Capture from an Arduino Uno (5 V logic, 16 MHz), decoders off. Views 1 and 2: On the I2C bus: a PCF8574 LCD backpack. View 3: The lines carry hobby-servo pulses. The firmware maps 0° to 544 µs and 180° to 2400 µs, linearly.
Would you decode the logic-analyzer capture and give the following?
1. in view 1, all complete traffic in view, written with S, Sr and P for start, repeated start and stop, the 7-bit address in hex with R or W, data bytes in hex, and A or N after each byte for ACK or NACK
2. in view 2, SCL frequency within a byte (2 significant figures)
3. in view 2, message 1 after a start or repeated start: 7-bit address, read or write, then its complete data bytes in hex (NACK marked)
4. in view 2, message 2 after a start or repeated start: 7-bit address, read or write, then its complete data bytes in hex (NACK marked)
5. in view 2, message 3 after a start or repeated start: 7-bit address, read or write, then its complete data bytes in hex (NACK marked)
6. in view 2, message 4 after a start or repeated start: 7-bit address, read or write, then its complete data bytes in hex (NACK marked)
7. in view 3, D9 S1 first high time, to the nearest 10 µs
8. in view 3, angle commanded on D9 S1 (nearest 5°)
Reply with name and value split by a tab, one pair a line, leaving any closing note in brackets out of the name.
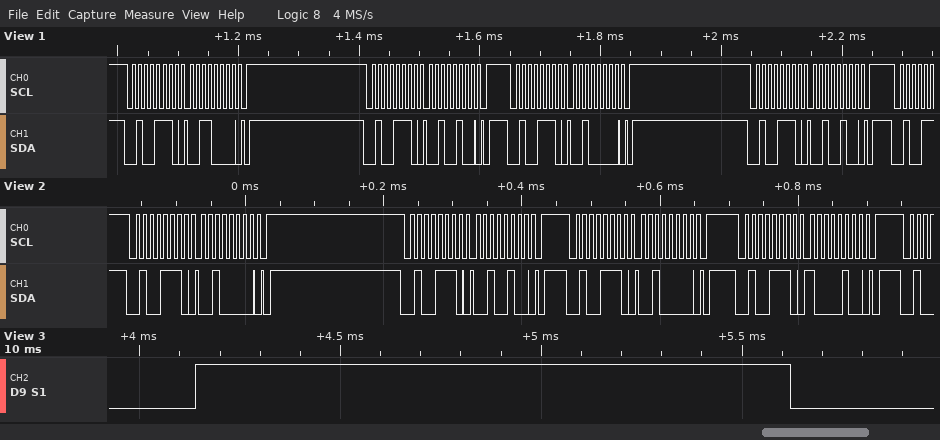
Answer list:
in view 1, all complete traffic in view, written with S, Sr and P for start, repeated start and stop, the 7-bit address in hex with R or W, data bytes in hex, and A or N after each byte for ACK or NACK	S 27W A 30 A P S 27W A 24 A P S 27W A 20 A P S 27W A 24 A P
in view 2, SCL frequency within a byte	100 kHz
in view 2, message 1 after a start or repeated start: 7-bit address, read or write, then its complete data bytes in hex	0x27 write: 20
in view 2, message 2 after a start or repeated start: 7-bit address, read or write, then its complete data bytes in hex	0x27 write: 24
in view 2, message 3 after a start or repeated start: 7-bit address, read or write, then its complete data bytes in hex	0x27 write: 20
in view 2, message 4 after a start or repeated start: 7-bit address, read or write, then its complete data bytes in hex	0x27 write: 84
in view 3, D9 S1 first high time, to the nearest 10 µs	1480 µs
in view 3, angle commanded on D9 S1	90°
